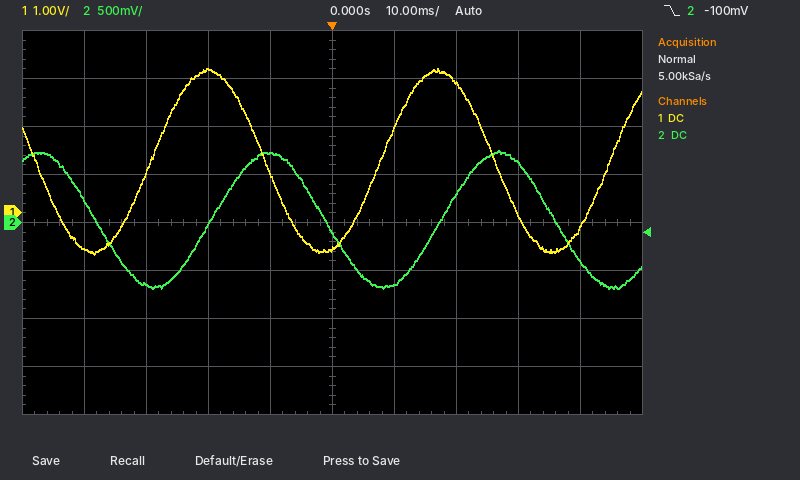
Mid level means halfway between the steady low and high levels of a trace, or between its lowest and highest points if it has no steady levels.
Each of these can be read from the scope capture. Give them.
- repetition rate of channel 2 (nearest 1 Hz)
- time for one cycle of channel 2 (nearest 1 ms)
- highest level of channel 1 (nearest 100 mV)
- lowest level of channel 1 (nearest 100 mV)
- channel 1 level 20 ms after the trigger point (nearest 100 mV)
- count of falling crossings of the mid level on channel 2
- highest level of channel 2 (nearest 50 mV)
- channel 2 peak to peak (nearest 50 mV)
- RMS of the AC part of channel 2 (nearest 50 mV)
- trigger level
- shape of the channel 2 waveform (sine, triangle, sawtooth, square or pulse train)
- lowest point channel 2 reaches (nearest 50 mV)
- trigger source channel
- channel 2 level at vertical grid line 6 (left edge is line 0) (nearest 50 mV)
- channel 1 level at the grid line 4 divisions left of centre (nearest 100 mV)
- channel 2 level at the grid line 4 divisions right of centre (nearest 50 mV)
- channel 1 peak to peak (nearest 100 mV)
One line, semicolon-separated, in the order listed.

27 Hz; 37 ms; 3.0 V; -900 mV; 2.7 V; 3; 750 mV; 1.45 V; 500 mV; -100 mV; sine; -700 mV; channel 2; -650 mV; -700 mV; -400 mV; 3.9 V
